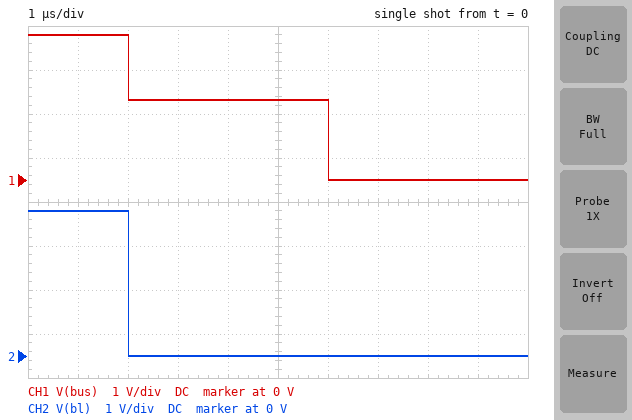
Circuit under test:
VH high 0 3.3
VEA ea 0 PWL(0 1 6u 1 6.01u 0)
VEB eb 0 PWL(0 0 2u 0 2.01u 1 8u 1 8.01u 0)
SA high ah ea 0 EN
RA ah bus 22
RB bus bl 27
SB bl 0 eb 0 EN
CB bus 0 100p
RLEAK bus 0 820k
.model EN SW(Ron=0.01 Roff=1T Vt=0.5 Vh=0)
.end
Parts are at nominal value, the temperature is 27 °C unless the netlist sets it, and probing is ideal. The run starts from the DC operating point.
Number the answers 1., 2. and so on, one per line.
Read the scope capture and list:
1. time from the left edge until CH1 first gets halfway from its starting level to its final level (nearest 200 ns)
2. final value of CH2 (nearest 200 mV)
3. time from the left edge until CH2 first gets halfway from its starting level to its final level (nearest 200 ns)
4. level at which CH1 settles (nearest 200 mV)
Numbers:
1. 6.0 µs
2. 0 V
3. 2.0 µs
4. 0 V
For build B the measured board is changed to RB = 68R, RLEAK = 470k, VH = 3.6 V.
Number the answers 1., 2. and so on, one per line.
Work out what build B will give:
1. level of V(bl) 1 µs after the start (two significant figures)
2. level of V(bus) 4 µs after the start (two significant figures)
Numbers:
1. 3.6 V
2. 2.7 V
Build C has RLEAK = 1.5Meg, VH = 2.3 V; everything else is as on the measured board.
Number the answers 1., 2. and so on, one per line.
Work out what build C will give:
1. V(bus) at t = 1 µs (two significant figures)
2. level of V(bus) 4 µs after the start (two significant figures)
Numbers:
1. 2.3 V
2. 1.3 V
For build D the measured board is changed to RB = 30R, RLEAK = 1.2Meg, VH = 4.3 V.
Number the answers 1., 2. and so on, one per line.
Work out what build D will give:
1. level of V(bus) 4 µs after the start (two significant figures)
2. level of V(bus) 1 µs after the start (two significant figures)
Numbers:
1. 2.5 V
2. 4.3 V
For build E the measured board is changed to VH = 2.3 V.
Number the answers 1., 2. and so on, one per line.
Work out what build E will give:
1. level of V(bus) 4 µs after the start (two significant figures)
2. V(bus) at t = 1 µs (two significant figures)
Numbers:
1. 1.3 V
2. 2.3 V
